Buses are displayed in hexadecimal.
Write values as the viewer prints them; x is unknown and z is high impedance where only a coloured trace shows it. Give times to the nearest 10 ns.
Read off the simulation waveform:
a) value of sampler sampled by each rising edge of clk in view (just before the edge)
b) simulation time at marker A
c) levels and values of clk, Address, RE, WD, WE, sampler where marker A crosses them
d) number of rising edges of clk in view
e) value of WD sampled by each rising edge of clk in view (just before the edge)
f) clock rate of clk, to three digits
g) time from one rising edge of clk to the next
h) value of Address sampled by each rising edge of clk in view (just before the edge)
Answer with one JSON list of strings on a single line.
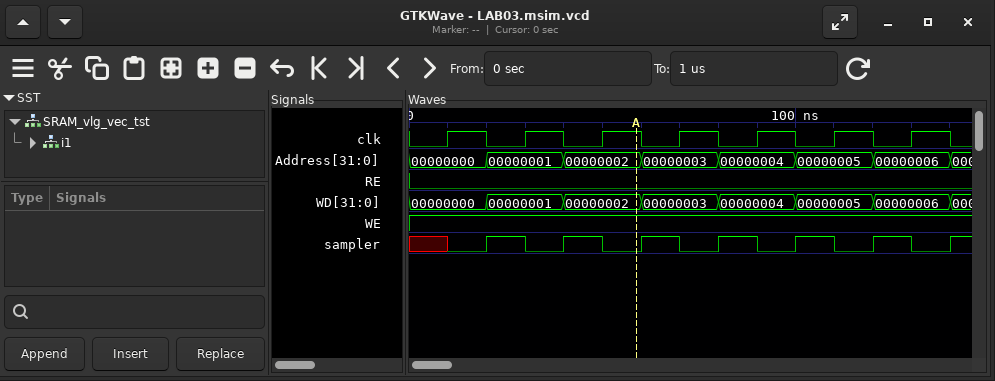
["x 1 1 1 1 1 1", "60 ns", "clk=1, Address=00000002, RE=0, WD=00000002, WE=1, sampler=0", "7", "00000000, 00000001, 00000002, 00000003, 00000004, 00000005, 00000006", "50.0 MHz", "20 ns", "00000000, 00000001, 00000002, 00000003, 00000004, 00000005, 00000006"]
